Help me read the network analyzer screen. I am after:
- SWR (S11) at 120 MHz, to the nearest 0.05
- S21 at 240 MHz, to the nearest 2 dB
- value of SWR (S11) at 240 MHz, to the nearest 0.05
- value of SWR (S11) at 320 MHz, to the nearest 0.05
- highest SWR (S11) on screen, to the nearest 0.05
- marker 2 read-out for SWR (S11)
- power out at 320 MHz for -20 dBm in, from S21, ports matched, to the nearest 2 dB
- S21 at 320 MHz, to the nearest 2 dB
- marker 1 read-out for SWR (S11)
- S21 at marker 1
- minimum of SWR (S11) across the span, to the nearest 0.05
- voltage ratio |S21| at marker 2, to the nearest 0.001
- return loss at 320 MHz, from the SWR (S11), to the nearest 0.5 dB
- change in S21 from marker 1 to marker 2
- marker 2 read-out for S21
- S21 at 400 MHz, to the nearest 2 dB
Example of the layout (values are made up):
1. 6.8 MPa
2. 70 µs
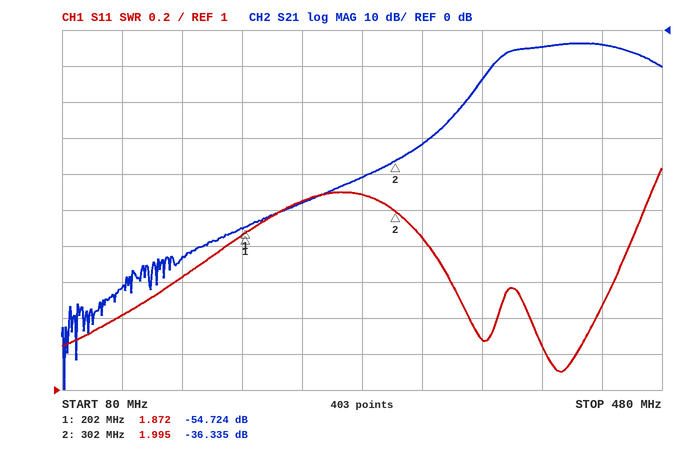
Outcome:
1. 1.40
2. -48 dB
3. 2.05
4. 1.85
5. 2.25
6. 1.995
7. -52 dBm
8. -32 dB
9. 1.872
10. -54.724 dB
11. 1.10
12. 0.015
13. 10.5 dB
14. 18.389 dB
15. -36.335 dB
16. -4 dB
